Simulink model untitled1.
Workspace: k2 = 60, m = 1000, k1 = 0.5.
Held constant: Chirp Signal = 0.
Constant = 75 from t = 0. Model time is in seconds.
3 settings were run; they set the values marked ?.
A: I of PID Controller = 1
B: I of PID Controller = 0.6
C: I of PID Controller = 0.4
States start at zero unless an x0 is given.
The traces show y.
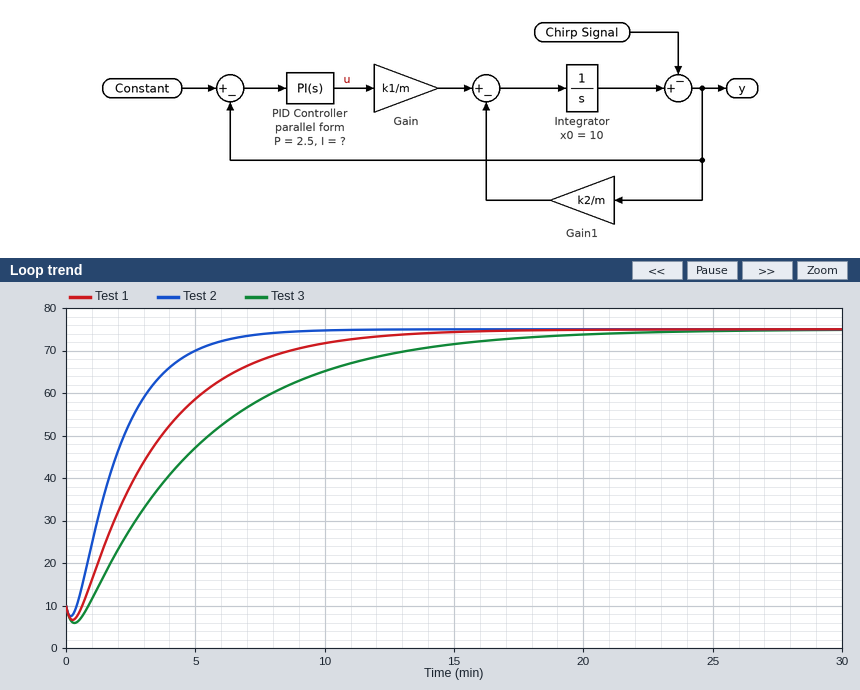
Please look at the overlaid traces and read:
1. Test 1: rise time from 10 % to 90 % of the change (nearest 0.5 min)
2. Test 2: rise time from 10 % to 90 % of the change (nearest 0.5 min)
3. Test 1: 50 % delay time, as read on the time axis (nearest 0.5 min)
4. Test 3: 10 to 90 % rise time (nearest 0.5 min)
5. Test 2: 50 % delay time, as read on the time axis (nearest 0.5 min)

7.0 min
4.0 min
3.0 min
10.5 min
2.0 min
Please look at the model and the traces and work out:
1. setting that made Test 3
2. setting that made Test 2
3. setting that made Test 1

C
A
B
